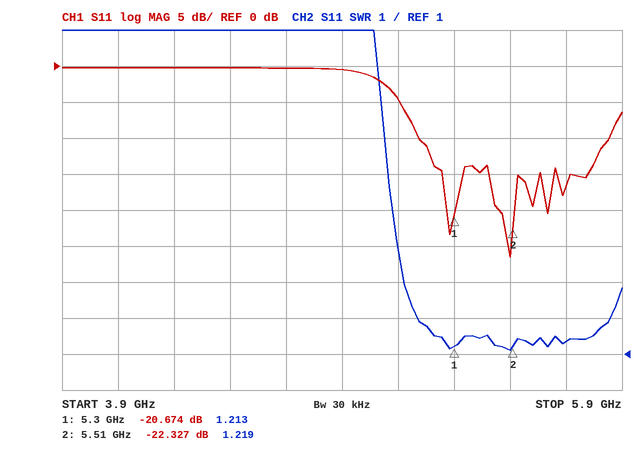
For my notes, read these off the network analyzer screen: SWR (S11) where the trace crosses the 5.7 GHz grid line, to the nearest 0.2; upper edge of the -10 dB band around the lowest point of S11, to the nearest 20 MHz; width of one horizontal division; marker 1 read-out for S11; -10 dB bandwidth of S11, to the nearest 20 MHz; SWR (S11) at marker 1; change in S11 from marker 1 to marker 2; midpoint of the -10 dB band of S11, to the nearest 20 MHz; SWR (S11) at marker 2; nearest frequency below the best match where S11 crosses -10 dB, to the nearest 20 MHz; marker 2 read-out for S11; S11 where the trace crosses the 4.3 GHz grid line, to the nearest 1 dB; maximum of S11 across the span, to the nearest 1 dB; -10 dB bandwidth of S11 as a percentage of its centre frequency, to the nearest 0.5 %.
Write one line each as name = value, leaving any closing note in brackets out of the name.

SWR (S11) where the trace crosses the 5.7 GHz grid line, to the nearest 0.2 = 1.4
upper edge of the -10 dB band around the lowest point of S11, to the nearest 20 MHz = 5.86 GHz
width of one horizontal division = 200 MHz
marker 1 read-out for S11 = -20.674 dB
-10 dB bandwidth of S11, to the nearest 20 MHz = 680 MHz
SWR (S11) at marker 1 = 1.213
change in S11 from marker 1 to marker 2 = -1.653 dB
midpoint of the -10 dB band of S11, to the nearest 20 MHz = 5.52 GHz
SWR (S11) at marker 2 = 1.219
nearest frequency below the best match where S11 crosses -10 dB, to the nearest 20 MHz = 5.18 GHz
marker 2 read-out for S11 = -22.327 dB
S11 where the trace crosses the 4.3 GHz grid line, to the nearest 1 dB = 0 dB
maximum of S11 across the span, to the nearest 1 dB = 0 dB
-10 dB bandwidth of S11 as a percentage of its centre frequency, to the nearest 0.5 % = 12.5 %
